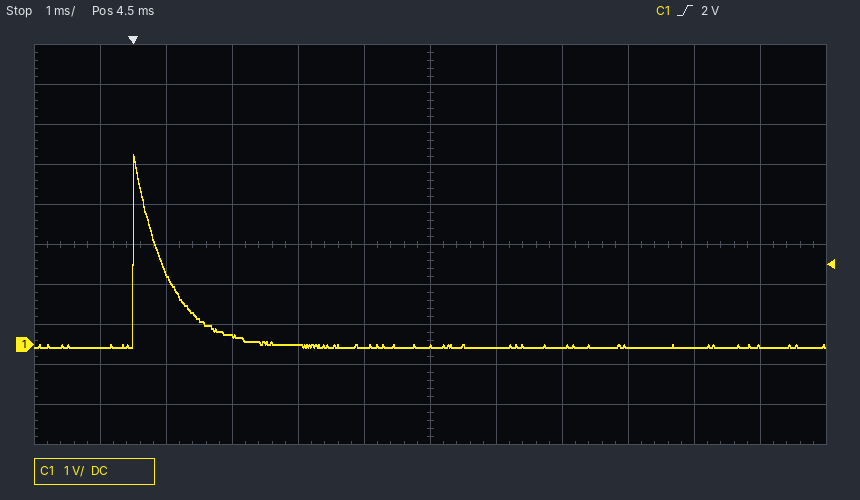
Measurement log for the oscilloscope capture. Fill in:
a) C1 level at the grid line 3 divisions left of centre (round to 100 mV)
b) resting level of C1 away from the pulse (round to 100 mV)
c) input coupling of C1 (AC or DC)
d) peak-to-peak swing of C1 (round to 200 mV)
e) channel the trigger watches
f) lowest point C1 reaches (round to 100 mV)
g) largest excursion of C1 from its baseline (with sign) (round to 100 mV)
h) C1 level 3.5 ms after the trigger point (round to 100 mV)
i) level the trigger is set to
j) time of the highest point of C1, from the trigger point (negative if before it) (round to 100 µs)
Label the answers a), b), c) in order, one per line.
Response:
a) 200 mV
b) -100 mV
c) DC
d) 4.8 V
e) C1
f) -100 mV
g) +4.8 V
h) -100 mV
i) 2 V
j) 0.0 ms
